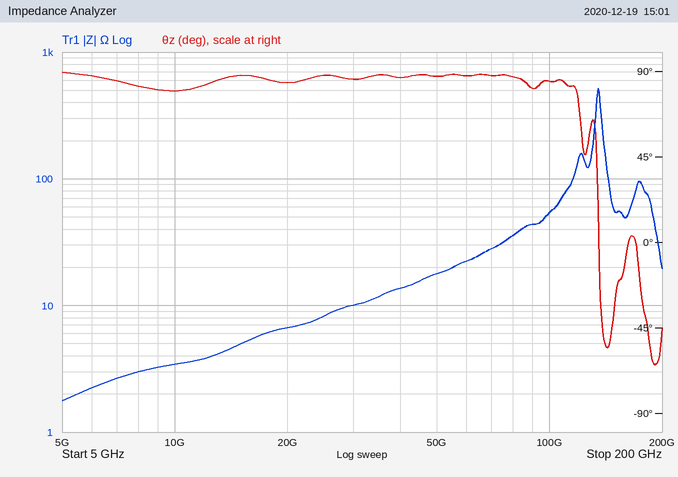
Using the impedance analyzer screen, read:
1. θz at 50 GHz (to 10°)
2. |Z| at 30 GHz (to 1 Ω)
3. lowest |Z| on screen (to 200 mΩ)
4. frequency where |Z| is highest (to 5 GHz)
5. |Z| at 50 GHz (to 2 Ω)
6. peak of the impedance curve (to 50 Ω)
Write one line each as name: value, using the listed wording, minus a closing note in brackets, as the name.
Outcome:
θz at 50 GHz: 90°
|Z| at 30 GHz: 10 Ω
lowest |Z| on screen: 1.8 Ω
frequency where |Z| is highest: 135 GHz
|Z| at 50 GHz: 18 Ω
peak of the impedance curve: 500 Ω
